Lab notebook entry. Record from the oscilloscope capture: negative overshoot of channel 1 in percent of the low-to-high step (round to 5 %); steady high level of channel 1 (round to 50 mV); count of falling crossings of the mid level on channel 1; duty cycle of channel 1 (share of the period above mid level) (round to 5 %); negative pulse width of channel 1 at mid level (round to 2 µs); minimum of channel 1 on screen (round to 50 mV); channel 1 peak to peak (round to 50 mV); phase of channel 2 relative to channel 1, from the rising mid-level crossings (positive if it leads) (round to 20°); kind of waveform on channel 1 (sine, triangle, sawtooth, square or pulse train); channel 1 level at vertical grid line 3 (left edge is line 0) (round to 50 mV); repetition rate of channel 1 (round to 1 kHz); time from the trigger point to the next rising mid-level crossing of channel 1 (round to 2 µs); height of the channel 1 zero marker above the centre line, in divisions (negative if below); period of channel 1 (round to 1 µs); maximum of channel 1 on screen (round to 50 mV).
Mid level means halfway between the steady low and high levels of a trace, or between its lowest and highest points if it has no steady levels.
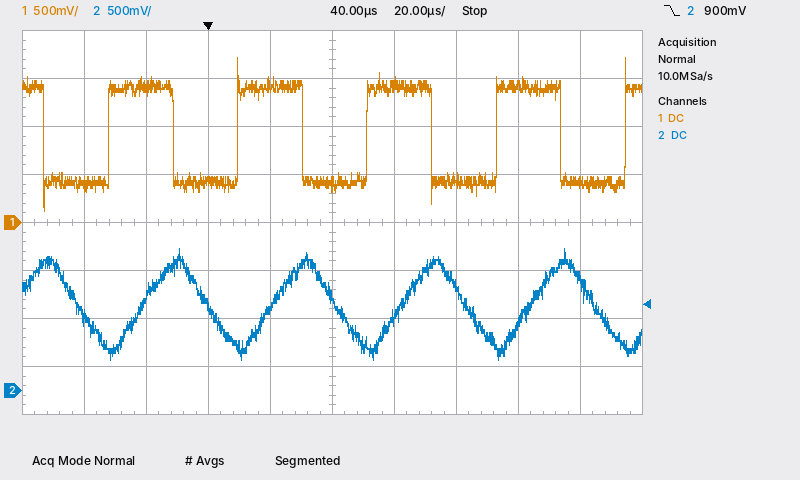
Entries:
30 %
1.40 V
5
50 %
20 µs
100 mV
1.60 V
-100°
square
450 mV
24 kHz
10 µs
0.0 div
42 µs
1.70 V
